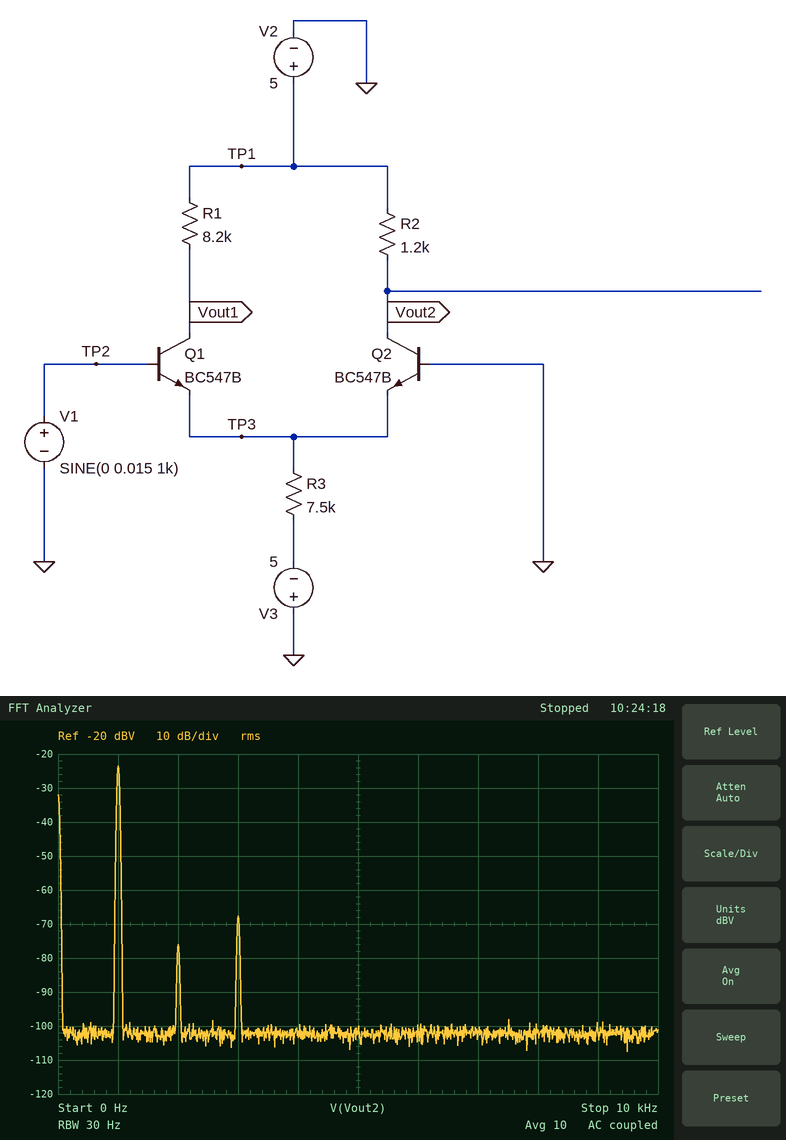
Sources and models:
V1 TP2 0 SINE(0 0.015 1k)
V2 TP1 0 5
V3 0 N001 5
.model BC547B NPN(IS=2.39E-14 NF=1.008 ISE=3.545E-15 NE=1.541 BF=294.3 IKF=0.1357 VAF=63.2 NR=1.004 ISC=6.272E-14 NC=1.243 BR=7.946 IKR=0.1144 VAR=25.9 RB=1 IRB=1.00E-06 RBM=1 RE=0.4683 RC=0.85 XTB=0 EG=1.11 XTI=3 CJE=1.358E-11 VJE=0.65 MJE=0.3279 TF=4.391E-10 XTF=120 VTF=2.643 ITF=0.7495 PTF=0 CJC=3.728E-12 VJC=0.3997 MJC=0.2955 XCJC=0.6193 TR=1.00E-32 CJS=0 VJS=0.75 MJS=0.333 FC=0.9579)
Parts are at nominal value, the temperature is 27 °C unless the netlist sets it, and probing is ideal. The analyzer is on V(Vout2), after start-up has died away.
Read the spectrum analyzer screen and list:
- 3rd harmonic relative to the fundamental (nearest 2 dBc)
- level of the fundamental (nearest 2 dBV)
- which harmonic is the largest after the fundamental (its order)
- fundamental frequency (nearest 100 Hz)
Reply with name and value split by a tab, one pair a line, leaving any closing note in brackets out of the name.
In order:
3rd harmonic relative to the fundamental	-44 dBc
level of the fundamental	-24 dBV
which harmonic is the largest after the fundamental	3
fundamental frequency	1.0 kHz
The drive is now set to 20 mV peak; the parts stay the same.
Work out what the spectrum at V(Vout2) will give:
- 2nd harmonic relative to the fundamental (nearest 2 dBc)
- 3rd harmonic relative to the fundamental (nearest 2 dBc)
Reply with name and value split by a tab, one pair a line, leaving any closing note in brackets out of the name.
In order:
2nd harmonic relative to the fundamental	-50 dBc
3rd harmonic relative to the fundamental	-40 dBc
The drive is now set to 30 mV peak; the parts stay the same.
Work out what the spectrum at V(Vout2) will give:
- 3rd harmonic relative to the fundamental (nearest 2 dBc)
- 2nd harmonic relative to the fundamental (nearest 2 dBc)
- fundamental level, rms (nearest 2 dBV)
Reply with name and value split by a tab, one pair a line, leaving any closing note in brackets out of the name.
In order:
3rd harmonic relative to the fundamental	-32 dBc
2nd harmonic relative to the fundamental	-48 dBc
fundamental level, rms	-18 dBV
